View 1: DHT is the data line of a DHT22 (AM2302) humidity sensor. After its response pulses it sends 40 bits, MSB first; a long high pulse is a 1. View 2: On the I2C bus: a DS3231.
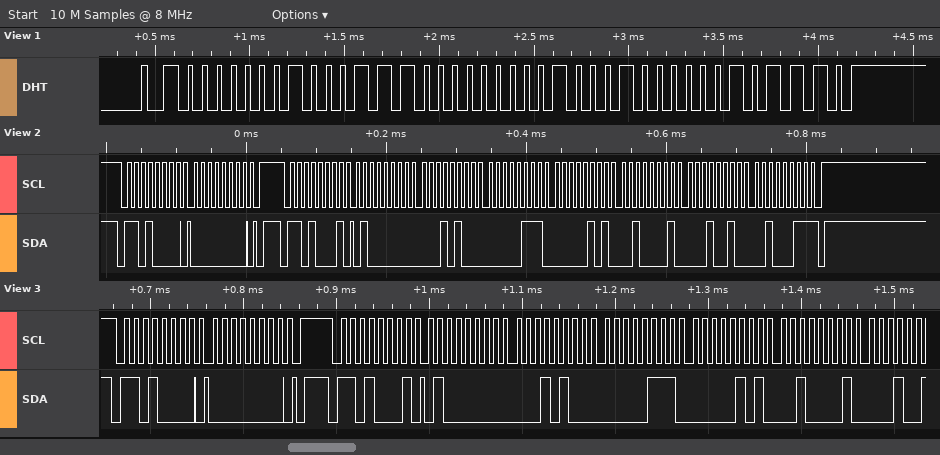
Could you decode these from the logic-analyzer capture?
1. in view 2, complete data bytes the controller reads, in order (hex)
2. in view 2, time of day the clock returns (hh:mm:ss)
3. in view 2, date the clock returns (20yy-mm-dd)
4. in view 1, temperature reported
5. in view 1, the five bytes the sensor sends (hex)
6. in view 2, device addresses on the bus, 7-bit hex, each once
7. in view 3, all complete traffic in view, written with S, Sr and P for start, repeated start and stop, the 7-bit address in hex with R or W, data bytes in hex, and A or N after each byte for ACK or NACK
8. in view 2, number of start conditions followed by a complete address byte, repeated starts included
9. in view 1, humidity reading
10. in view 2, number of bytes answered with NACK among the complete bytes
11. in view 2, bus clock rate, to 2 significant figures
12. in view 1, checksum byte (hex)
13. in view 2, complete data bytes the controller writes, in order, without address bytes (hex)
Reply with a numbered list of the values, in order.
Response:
1. 40 14 07 05 21 12 23
2. 07:14:40
3. 2023-12-21
4. 27.2 °C
5. 01 1C 01 10 2E
6. 0x68
7. S 68W A 00 A P S 68R A 40 A 14 A 07 A 05 A 21 A
8. 2
9. 28.4 %
10. 1
11. 100 kHz
12. 0x2E
13. 00
